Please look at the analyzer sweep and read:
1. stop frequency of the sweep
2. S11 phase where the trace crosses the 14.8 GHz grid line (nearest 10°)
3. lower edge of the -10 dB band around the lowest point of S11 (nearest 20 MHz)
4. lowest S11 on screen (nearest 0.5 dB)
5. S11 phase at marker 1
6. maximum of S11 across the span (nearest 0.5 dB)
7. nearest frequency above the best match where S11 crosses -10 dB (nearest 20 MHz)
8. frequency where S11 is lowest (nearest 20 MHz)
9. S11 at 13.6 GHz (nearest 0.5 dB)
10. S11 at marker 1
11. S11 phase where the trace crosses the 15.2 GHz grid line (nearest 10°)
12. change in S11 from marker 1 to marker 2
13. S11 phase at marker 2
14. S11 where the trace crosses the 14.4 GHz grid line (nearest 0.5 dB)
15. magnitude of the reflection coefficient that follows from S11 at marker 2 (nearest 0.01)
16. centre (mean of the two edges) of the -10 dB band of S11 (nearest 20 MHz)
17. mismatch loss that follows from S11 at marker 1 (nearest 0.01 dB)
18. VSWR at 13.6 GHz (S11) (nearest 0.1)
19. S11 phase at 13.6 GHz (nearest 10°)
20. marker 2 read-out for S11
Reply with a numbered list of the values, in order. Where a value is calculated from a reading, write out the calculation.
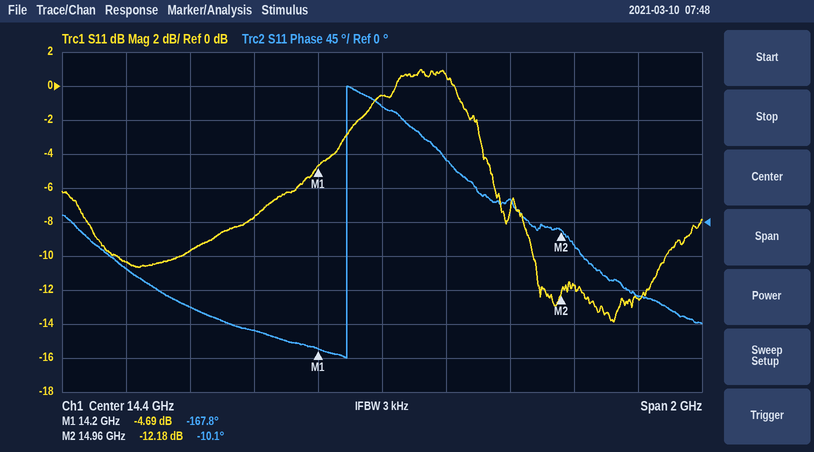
1. 15.4 GHz
2. 30°
3. 14.88 GHz
4. -14.0 dB
5. -167.8°
6. 1.0 dB
7. 15.28 GHz
8. 15.12 GHz
9. -10.5 dB
10. -4.69 dB
11. -100°
12. -12.18 − (-4.69) = -7.49 dB
13. -10.1°
14. -0.5 dB
15. 10^(-12.18/20) ≈ 0.25
16. 15.08 GHz
17. −10 log10(1 − 10^(-4.69/10)) ≈ 1.80 dB
18. |Γ| = 10^(-10.5/20) = 0.2985; VSWR = (1 + 0.2985)/(1 − 0.2985) ≈ 1.9
19. -60°
20. -12.18 dB
